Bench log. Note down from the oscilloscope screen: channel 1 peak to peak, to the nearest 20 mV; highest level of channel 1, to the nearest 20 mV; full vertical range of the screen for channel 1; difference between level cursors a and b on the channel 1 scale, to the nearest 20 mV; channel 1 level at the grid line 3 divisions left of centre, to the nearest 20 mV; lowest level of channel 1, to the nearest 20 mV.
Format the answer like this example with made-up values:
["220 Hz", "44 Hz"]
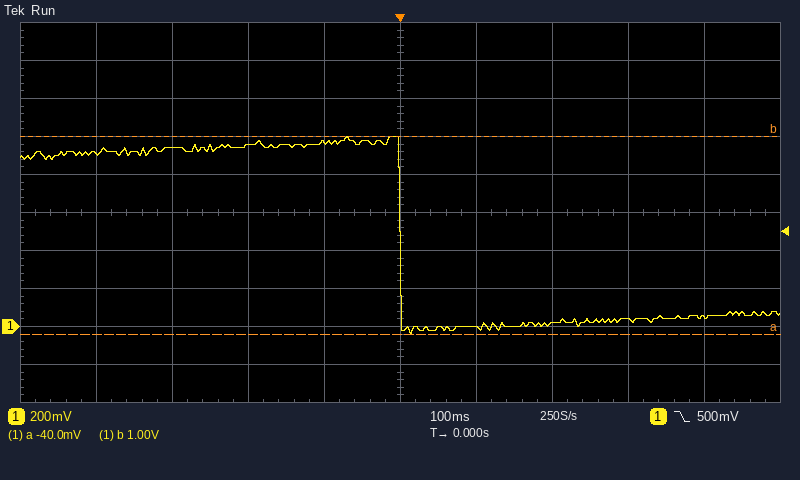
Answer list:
["1.04 V", "1.00 V", "2 V", "1.04 V", "940 mV", "-40 mV"]
